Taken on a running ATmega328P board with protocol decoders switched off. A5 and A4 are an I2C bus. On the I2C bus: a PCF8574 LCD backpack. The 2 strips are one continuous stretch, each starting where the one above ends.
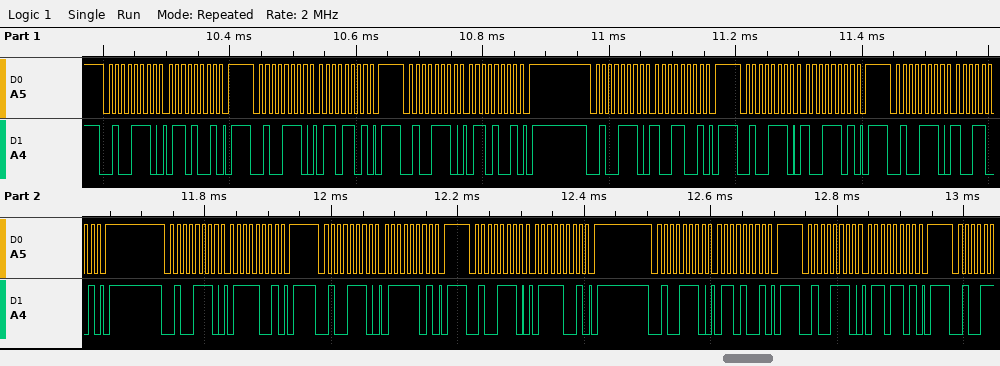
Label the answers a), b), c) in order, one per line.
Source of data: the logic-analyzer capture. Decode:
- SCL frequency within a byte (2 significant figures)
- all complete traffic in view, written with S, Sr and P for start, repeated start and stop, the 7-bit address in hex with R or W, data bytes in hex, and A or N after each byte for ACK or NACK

a) 100 kHz
b) S 27W A 69 A P S 27W A 6D A P S 27W A 69 A P S 27W A 99 A P S 27W A 9D A P S 27W A 99 A P S 27W A 79 A P S 27W A 7D A P S 27W A 79 A P S 27W A 69 A P S 27W A 6D A P
